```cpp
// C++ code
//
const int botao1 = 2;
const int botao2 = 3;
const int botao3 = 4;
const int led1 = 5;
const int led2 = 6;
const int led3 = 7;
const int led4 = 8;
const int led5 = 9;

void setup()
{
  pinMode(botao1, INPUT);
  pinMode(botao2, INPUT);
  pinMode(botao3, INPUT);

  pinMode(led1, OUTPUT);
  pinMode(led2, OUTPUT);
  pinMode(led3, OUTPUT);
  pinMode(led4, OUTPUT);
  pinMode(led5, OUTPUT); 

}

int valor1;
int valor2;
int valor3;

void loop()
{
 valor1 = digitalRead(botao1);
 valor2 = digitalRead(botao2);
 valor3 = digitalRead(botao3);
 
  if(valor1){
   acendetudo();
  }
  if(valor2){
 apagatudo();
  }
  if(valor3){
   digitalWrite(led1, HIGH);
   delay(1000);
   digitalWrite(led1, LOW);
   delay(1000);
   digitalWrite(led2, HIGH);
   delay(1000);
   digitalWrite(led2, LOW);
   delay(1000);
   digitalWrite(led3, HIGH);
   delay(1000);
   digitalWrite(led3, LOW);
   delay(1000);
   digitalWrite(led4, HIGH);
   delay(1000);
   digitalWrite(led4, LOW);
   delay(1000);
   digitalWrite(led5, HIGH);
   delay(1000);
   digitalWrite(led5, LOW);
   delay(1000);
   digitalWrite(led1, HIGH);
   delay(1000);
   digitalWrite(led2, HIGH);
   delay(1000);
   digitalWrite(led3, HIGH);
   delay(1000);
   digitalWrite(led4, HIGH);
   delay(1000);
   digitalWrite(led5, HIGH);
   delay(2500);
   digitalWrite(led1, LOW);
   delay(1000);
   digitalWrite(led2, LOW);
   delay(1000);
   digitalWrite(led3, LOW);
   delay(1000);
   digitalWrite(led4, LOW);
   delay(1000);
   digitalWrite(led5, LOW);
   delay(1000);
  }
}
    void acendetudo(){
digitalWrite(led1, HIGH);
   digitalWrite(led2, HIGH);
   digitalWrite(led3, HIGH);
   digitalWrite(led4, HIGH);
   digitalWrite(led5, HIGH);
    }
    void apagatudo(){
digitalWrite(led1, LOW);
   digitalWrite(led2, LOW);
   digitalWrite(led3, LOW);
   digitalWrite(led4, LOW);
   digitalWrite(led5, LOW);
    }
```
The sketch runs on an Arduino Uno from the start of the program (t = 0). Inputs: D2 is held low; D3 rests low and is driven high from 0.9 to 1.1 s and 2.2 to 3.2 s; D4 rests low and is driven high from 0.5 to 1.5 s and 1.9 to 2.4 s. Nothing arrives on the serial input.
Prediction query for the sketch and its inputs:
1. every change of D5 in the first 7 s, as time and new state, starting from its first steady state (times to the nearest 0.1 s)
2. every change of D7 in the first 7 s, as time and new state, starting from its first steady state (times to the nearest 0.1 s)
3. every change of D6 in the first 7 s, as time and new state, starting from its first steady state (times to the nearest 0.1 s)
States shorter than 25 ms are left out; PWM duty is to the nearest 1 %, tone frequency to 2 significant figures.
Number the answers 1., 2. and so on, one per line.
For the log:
1. 0 s low; 0.5 s high; 1.5 s low
2. 0 s low; 4.5 s high; 5.5 s low
3. 0 s low; 2.5 s high; 3.5 s low
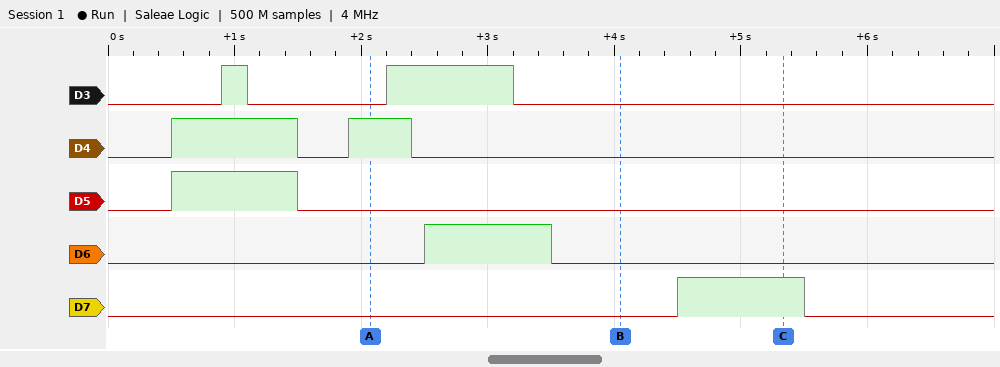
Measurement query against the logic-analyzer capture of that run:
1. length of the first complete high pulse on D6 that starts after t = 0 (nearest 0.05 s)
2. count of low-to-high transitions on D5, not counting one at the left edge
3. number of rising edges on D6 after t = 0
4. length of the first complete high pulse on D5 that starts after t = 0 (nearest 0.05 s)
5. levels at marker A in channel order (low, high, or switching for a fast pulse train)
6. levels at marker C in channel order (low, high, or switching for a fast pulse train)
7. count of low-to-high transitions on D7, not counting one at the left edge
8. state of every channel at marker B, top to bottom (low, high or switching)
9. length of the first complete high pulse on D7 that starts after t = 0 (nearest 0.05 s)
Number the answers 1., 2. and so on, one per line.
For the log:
1. 1.00 s
2. 1
3. 1
4. 1.00 s
5. D3 low, D4 high, D5 low, D6 low, D7 low
6. D3 low, D4 low, D5 low, D6 low, D7 high
7. 1
8. D3 low, D4 low, D5 low, D6 low, D7 low
9. 1.00 s
